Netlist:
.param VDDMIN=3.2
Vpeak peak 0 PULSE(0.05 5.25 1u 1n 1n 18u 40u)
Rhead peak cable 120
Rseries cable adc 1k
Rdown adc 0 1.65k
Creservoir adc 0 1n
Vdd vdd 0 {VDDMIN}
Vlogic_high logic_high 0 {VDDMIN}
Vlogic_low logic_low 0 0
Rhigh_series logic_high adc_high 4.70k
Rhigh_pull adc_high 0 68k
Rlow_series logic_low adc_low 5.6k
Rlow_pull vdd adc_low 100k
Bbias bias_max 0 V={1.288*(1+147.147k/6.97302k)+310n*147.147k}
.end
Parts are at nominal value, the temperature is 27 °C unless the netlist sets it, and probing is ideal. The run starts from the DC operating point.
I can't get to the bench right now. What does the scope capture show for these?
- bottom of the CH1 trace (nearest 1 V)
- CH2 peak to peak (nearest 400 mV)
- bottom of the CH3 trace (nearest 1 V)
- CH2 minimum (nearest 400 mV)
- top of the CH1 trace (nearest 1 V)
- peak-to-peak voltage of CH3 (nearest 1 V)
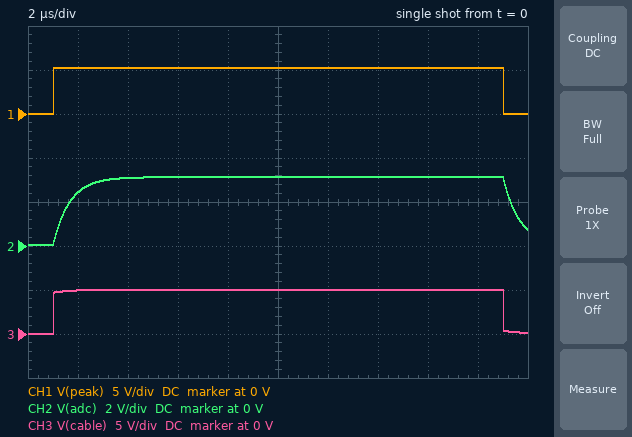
0 V
3.2 V
0 V
0 V
5 V
5 V
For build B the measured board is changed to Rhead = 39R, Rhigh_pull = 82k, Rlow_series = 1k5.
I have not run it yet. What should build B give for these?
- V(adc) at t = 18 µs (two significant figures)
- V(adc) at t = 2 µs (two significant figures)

3.2 V
2.6 V
